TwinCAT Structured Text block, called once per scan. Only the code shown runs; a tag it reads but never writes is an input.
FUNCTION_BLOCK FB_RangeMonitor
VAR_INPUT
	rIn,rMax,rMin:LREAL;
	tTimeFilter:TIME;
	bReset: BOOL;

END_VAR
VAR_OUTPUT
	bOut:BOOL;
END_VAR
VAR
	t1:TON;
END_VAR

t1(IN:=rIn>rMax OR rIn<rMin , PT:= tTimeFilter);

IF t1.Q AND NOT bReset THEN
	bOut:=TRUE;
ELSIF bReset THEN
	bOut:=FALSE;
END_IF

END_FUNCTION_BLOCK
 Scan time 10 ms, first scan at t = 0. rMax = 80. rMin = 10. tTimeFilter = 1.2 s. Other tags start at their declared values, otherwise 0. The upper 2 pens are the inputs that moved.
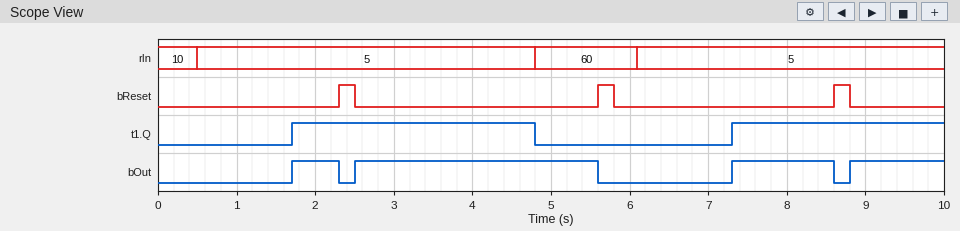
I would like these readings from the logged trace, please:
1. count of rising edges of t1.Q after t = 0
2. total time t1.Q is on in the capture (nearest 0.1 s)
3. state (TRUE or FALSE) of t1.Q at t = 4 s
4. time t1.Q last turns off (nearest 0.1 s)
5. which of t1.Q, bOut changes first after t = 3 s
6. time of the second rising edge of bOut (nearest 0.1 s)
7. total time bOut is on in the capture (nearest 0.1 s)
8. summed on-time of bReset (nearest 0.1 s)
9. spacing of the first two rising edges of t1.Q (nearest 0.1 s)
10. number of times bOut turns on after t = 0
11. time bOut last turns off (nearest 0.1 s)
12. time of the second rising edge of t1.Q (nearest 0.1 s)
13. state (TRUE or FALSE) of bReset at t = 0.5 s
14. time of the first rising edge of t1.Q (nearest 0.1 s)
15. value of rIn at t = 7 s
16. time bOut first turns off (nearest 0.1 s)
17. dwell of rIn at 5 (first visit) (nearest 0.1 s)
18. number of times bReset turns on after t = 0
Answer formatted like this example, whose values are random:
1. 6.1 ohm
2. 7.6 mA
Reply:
1. 2
2. 5.8 s
3. TRUE
4. 4.8 s
5. t1.Q
6. 2.5 s
7. 6.2 s
8. 0.6 s
9. 5.6 s
10. 4
11. 8.6 s
12. 7.3 s
13. FALSE
14. 1.7 s
15. 5
16. 2.3 s
17. 4.3 s
18. 3
